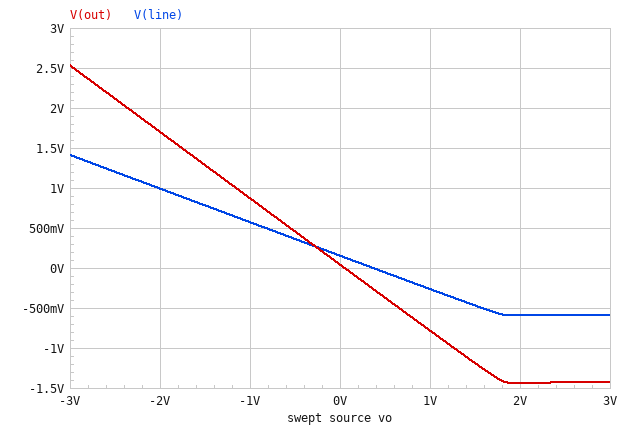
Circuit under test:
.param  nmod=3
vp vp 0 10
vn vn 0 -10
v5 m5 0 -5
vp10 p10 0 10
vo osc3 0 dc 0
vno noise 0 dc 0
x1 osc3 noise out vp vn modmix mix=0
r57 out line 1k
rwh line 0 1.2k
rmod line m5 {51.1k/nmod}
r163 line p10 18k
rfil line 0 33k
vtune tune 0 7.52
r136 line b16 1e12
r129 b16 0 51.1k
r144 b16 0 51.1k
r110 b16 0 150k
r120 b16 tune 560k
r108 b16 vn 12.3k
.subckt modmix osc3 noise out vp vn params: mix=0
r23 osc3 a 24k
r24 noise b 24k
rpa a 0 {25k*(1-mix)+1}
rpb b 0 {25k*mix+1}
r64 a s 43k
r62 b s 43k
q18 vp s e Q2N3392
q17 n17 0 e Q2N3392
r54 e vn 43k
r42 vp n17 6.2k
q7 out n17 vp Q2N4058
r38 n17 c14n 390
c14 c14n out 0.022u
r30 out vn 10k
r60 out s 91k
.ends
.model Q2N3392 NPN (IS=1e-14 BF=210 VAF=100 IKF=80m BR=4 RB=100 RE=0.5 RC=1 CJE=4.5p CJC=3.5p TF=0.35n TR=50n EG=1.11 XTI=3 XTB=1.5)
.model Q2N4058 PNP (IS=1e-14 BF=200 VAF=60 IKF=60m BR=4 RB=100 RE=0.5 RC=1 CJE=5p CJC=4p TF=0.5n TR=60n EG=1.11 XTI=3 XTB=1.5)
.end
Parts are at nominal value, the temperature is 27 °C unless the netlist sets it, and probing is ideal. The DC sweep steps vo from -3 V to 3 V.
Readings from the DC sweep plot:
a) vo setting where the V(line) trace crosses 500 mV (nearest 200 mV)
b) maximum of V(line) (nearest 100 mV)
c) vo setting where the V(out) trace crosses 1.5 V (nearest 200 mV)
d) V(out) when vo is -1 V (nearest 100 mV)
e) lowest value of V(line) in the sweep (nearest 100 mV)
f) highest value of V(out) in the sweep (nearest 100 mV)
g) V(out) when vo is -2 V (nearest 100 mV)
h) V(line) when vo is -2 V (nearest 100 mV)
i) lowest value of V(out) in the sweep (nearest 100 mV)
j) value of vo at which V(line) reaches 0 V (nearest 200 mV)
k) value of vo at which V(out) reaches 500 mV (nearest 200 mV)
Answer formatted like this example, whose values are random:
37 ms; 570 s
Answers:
-800 mV; 1.4 V; -1.8 V; 900 mV; -600 mV; 2.5 V; 1.7 V; 1.0 V; -1.4 V; 400 mV; -600 mV
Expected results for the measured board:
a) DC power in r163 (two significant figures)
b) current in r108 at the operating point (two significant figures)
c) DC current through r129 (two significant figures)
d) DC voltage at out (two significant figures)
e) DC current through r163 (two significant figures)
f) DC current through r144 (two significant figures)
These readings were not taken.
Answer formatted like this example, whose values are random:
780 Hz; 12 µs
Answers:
5.4 mW; 310 µA; 120 µA; 43 mV; 550 µA; 120 µA
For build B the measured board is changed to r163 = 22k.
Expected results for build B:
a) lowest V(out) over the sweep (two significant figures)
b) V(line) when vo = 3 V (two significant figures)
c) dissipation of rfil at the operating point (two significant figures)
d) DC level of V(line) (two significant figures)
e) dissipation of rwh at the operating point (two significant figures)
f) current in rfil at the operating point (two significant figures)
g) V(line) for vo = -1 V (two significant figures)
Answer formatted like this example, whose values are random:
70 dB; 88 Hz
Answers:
-1.5 V; -690 mV; 320 nW; 100 mV; 8.8 µW; 3.1 µA; 520 mV
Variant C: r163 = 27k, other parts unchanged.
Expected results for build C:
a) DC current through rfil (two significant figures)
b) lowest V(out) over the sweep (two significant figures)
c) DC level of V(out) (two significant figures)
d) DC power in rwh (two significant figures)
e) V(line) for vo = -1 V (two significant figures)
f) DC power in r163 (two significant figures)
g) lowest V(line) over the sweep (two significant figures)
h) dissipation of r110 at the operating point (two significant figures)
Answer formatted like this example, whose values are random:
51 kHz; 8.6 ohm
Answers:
1.8 µA; -1.6 V; 40 mV; 3.0 µW; 480 mV; 3.7 mW; -780 mV; 260 µW
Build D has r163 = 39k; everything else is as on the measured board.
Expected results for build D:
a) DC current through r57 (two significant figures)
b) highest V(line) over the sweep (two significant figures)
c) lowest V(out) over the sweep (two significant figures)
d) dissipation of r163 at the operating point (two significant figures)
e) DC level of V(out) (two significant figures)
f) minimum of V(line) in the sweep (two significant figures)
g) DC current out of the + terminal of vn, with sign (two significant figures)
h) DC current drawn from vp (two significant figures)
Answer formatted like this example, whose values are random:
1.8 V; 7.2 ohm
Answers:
38 µA; 1.3 V; -1.7 V; 2.6 mW; 39 mV; -890 mV; -1.5 mA; 1.3 mA
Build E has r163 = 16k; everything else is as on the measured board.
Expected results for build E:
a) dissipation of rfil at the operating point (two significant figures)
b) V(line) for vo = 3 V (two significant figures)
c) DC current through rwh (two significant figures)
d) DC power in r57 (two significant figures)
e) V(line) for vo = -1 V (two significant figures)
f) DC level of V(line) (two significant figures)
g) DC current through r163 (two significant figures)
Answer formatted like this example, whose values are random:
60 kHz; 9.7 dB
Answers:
1.1 µW; -520 mV; 160 µA; 21 µW; 610 mV; 190 mV; 610 µA
